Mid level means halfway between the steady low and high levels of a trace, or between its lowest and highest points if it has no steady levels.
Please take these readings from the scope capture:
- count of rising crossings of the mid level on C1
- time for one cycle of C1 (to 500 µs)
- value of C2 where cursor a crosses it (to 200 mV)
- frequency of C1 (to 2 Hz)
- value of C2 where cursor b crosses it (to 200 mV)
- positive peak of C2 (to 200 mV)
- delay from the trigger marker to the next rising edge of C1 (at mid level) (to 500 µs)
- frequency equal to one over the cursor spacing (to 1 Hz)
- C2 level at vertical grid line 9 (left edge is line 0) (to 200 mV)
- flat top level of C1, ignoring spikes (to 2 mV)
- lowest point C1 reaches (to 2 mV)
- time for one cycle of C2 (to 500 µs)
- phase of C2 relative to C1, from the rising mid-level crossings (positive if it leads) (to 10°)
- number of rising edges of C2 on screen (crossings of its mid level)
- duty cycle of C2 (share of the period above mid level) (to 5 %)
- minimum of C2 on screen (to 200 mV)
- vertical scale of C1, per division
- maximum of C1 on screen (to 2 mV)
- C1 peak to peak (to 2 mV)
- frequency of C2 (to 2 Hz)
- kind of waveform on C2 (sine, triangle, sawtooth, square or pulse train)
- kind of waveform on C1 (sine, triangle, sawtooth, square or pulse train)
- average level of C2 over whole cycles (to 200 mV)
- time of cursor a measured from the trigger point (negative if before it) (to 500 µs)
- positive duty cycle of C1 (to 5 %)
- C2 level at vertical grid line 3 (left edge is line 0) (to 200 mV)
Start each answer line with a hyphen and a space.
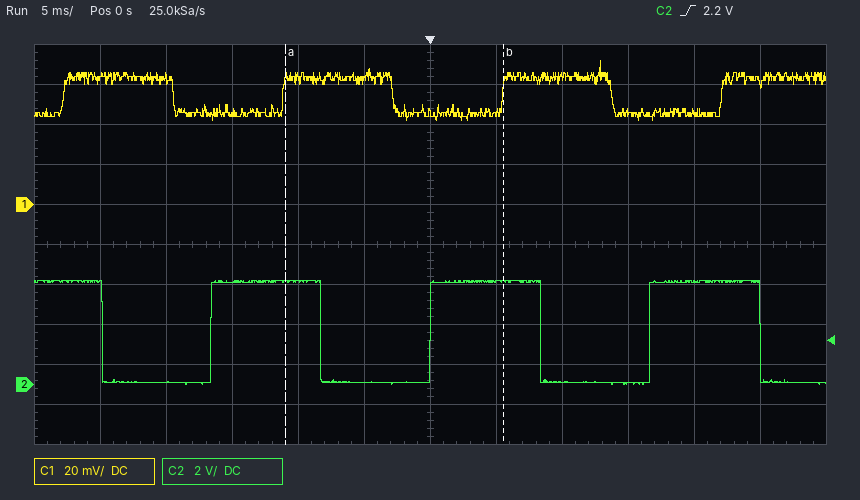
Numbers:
- 4
- 16.5 ms
- 5.2 V
- 60 Hz
- 5.2 V
- 5.2 V
- 5.5 ms
- 61 Hz
- 0.0 V
- 64 mV
- 42 mV
- 16.5 ms
- +120°
- 3
- 50 %
- 0.0 V
- 20 mV
- 72 mV
- 30 mV
- 60 Hz
- square
- square
- 2.6 V
- -11.0 ms
- 50 %
- 5.2 V
